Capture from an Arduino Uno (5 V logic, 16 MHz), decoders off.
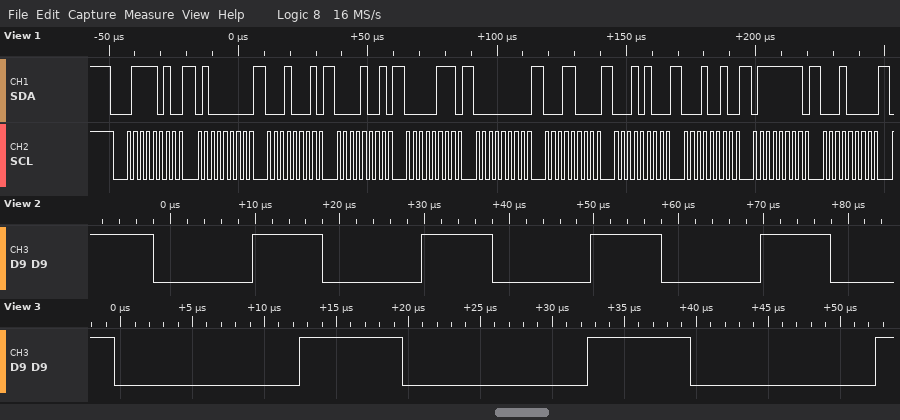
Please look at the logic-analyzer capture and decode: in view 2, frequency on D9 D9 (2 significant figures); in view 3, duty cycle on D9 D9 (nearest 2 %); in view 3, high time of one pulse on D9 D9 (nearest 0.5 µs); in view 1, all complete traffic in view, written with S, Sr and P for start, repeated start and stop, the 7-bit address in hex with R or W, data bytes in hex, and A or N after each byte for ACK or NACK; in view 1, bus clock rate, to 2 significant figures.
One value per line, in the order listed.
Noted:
50 kHz
36 %
7.0 µs
S 3DW A 40 A 11 A 09 A 07 A 00 A 18 A 14 A 12 A 7F A 10 A
400 kHz
